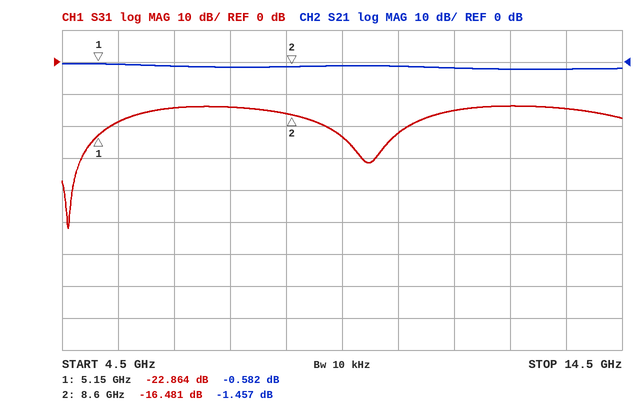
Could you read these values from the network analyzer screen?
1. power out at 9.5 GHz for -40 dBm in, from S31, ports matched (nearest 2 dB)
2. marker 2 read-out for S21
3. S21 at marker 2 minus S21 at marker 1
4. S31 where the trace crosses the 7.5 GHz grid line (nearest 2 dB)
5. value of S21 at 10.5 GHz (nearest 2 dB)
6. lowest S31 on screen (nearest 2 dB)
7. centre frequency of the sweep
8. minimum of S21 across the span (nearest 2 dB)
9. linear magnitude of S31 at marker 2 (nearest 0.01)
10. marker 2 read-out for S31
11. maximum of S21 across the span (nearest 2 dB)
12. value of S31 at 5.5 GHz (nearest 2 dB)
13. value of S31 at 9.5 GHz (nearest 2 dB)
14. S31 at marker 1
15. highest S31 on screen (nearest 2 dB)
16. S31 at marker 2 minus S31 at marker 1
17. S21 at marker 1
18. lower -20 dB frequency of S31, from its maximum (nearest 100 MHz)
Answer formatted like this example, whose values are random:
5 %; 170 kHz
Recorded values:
-64 dBm; -1.457 dB; -0.875 dB; -14 dB; -2 dB; -52 dB; 9.5 GHz; -2 dB; 0.15; -16.481 dB; 0 dB; -18 dB; -24 dB; -22.864 dB; -14 dB; 6.383 dB; -0.582 dB; 4.8 GHz
